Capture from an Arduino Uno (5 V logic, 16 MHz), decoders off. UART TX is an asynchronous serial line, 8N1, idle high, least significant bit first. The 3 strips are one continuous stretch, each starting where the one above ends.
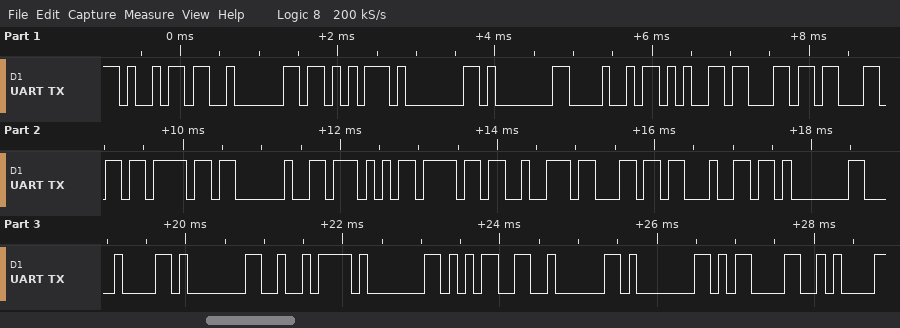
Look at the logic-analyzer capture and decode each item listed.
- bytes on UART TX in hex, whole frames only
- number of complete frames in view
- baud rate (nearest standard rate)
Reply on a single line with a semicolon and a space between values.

0x69 0x02 0xAB 0x01 0x01 0x48 0x65 0x6C 0x6C 0x6F 0x20 0x57 0x6F 0x72 0x6C 0x64 0x01 0x08 0x01 0xD2 0x01 0x35 0x02 0x01 0x0D 0x0A; 26; 9600 baud
